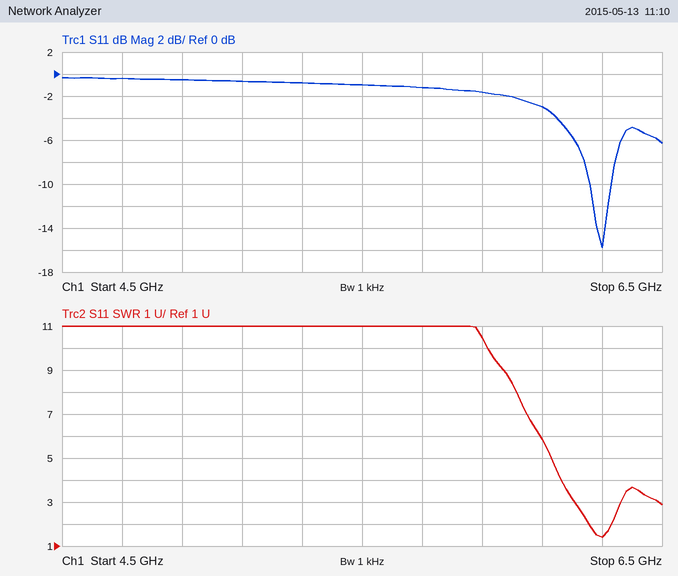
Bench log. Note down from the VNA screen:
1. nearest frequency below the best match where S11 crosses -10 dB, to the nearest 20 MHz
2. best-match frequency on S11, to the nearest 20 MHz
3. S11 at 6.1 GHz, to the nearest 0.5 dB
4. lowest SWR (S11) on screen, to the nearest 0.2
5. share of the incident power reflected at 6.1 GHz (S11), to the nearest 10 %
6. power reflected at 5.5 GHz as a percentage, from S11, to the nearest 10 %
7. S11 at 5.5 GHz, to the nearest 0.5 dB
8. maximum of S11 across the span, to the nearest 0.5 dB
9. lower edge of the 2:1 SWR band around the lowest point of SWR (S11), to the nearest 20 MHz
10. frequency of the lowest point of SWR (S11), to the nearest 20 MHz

6.26 GHz
6.30 GHz
-3.0 dB
1.4
50 %
80 %
-1.0 dB
-0.5 dB
6.26 GHz
6.30 GHz
